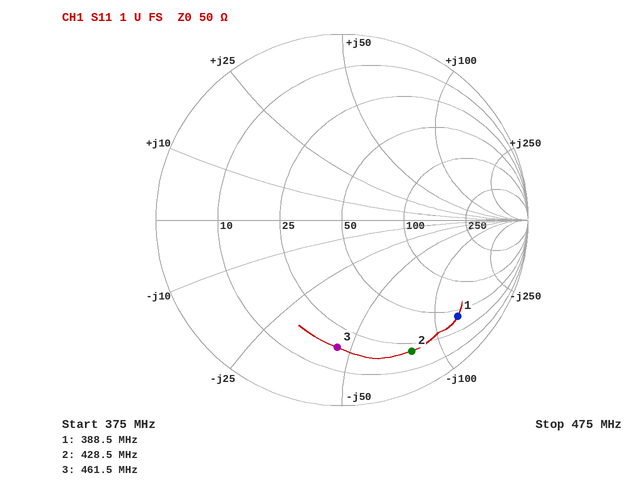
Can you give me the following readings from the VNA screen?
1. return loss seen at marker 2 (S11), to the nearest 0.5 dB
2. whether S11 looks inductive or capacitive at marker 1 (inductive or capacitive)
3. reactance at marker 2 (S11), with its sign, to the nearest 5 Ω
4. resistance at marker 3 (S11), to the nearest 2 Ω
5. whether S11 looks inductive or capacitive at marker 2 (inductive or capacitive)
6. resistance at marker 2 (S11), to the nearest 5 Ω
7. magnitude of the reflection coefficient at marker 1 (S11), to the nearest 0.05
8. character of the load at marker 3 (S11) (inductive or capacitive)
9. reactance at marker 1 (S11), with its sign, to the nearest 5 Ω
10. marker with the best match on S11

2.0 dB
capacitive
-80 Ω
18 Ω
capacitive
20 Ω
0.80
capacitive
-125 Ω
marker 3
